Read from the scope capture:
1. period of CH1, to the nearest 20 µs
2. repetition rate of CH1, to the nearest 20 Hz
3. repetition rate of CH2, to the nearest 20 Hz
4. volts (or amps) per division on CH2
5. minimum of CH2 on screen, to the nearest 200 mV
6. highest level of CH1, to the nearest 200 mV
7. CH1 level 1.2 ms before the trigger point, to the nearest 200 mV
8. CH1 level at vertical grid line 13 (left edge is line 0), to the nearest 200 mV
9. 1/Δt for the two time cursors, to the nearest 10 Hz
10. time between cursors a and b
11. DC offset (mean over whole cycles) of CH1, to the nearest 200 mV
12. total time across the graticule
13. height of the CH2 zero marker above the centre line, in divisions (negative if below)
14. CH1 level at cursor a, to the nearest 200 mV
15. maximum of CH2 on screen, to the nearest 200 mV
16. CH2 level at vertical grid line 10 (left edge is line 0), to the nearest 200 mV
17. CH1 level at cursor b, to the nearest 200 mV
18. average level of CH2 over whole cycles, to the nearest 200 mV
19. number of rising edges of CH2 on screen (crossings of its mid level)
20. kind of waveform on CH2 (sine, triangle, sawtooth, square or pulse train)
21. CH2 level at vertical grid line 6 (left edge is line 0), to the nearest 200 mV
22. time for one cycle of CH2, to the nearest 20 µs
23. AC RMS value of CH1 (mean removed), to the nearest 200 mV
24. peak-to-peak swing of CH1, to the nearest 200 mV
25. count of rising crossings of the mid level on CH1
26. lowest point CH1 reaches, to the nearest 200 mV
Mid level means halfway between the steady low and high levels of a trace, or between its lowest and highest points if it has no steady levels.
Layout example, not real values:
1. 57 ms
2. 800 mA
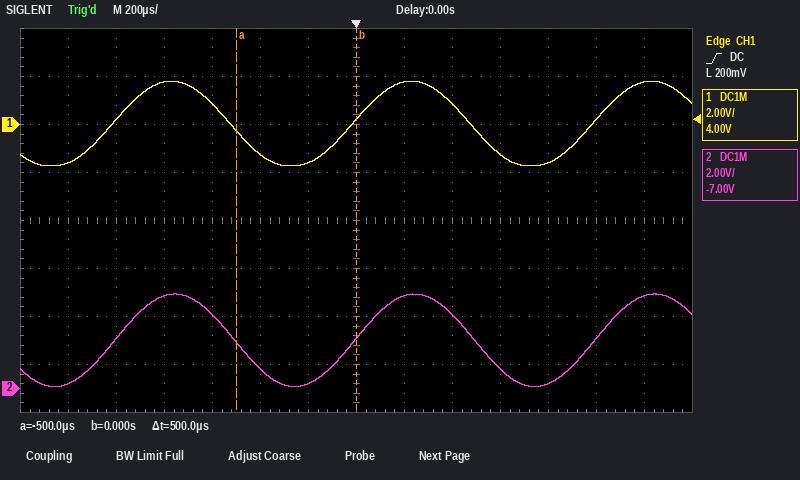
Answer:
1. 1.00 ms
2. 1.00 kHz
3. 1.00 kHz
4. 2 V
5. 0.0 V
6. 1.8 V
7. -1.6 V
8. 1.8 V
9. 2.00 kHz
10. 500 µs
11. 0.0 V
12. 2.8 ms
13. -3.5 div
14. -200 mV
15. 4.0 V
16. 800 mV
17. 200 mV
18. 2.0 V
19. 3
20. sine
21. 200 mV
22. 1.00 ms
23. 1.2 V
24. 3.6 V
25. 3
26. -1.8 V
